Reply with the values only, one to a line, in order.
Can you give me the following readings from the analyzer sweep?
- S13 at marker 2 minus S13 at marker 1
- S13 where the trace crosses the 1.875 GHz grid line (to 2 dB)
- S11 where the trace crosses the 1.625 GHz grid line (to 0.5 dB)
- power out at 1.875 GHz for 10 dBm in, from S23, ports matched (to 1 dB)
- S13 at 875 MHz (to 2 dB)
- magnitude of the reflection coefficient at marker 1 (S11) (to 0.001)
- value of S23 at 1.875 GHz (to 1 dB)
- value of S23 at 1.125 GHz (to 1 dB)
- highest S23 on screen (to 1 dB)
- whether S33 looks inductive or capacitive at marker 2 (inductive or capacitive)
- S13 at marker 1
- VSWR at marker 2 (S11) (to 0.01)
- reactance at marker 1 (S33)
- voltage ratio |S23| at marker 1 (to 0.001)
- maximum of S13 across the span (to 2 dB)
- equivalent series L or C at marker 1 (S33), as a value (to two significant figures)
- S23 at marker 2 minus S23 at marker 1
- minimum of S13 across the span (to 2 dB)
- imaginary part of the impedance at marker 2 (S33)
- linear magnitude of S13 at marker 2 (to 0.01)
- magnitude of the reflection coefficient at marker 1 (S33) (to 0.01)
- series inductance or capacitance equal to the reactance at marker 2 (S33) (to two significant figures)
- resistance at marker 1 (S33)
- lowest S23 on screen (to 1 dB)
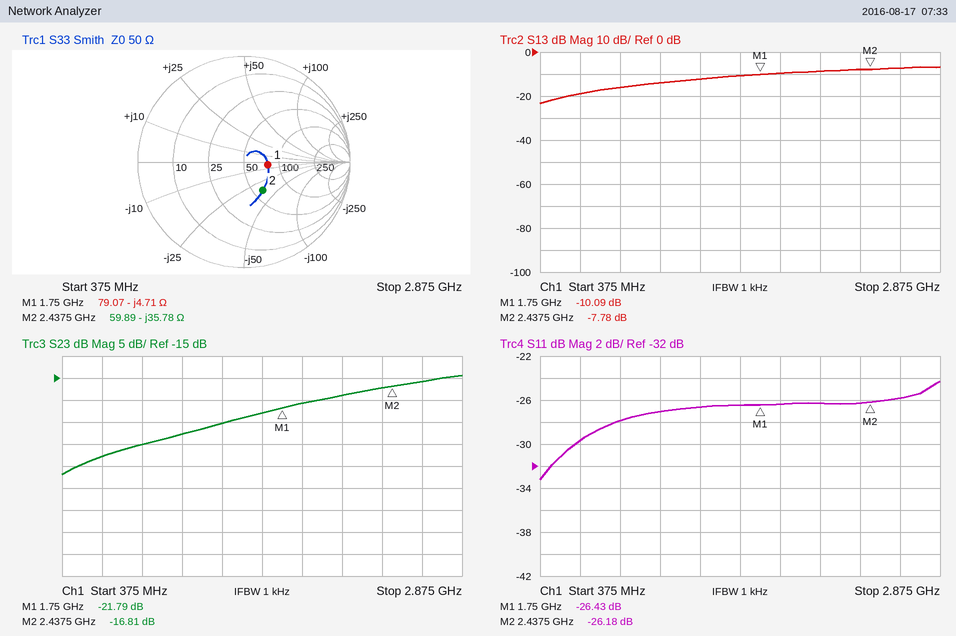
2.31 dB
-10 dB
-26.5 dB
-11 dBm
-16 dB
0.048
-21 dB
-28 dB
-14 dB
capacitive
-10.09 dB
1.10
-4.71 Ω
0.081
-6 dB
19 pF
4.98 dB
-24 dB
-35.78 Ω
0.41
0.23
1.8 pF
79.07 Ω
-37 dB
